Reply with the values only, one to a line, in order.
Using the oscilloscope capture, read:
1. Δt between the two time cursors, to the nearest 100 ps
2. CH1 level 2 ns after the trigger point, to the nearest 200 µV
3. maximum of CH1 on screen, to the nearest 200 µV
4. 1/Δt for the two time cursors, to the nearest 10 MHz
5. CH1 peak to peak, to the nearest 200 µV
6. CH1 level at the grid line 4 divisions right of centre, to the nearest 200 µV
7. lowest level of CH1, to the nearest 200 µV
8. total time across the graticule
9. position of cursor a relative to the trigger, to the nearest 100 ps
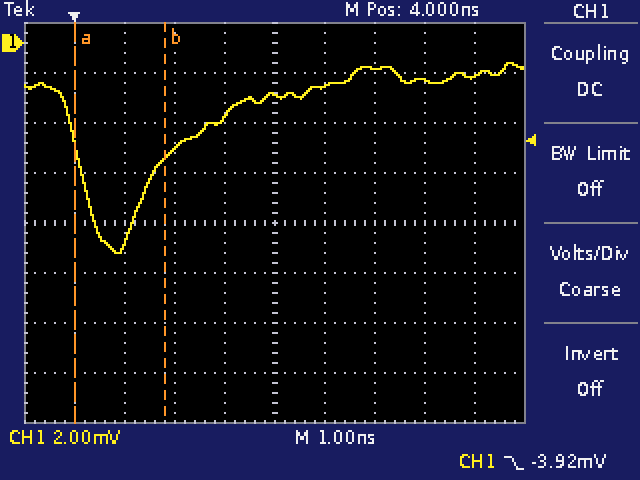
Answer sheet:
1.8 ns
-4.2 mV
-800 µV
560 MHz
7.6 mV
-1.4 mV
-8.4 mV
10 ns
0.0 ns
